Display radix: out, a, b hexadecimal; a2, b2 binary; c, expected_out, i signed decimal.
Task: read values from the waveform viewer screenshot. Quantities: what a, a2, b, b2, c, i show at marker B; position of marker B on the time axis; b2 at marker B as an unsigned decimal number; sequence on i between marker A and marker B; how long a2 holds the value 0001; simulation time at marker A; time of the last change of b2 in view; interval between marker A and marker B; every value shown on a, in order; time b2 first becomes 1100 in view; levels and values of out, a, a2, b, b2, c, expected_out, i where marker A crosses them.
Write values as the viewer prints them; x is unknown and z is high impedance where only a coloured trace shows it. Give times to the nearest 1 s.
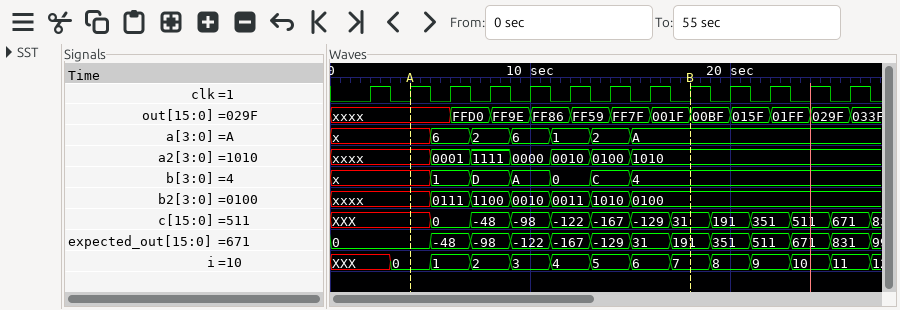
a=A, a2=1010, b=4, b2=0100, c=31, i=7
18 s
4
0, 1, 2, 3, 4, 5, 6, 7
2 s
4 s
15 s
14 s
x, 6, 2, 6, 1, 2, A
7 s
out=xxxx, a=x, a2=xxxx, b=x, b2=xxxx, c=XXX, expected_out=0, i=0
